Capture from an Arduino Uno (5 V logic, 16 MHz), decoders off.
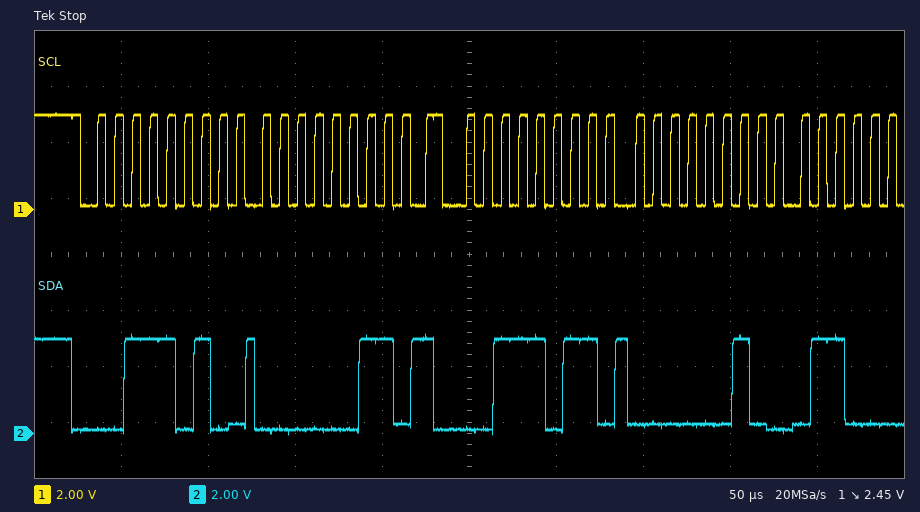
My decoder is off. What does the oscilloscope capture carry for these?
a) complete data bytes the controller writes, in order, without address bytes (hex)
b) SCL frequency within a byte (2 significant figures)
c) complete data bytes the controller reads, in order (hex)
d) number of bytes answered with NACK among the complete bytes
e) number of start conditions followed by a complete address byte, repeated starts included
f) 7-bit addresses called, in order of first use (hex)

03
100 kHz
02
0
2
0x1D
